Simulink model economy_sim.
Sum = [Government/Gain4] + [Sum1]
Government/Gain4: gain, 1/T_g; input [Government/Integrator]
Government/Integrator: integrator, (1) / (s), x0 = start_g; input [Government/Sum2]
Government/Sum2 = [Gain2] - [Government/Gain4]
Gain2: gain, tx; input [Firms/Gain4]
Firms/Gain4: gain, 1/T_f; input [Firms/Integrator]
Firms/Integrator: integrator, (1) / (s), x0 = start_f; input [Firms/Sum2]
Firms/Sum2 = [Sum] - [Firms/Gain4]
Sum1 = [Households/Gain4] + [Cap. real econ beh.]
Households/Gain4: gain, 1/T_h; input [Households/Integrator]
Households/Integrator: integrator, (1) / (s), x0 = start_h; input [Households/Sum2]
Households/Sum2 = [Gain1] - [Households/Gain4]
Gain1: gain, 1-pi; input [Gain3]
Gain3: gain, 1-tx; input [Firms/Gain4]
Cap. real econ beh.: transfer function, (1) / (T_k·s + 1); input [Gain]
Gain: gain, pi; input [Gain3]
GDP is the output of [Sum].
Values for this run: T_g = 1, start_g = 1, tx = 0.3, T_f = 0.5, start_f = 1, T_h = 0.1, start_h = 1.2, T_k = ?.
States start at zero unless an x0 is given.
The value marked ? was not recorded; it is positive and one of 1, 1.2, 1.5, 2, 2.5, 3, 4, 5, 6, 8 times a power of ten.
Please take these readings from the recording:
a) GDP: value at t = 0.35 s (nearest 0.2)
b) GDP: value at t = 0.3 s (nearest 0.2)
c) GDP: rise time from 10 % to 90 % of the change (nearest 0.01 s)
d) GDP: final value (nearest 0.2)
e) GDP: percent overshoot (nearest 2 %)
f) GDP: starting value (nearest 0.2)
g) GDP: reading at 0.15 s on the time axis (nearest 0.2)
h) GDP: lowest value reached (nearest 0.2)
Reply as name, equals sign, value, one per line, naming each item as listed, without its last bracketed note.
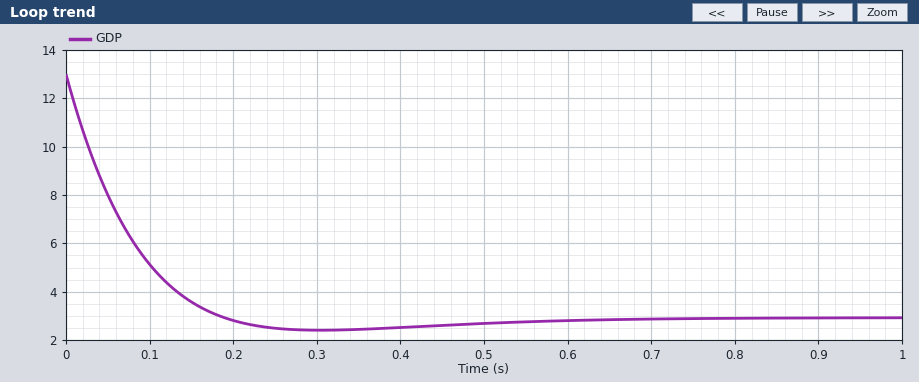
GDP: value at t = 0.35 s = 2.4
GDP: value at t = 0.3 s = 2.4
GDP: rise time from 10 % to 90 % of the change = 0.13 s
GDP: final value = 3.0
GDP: percent overshoot = 6 %
GDP: starting value = 13.0
GDP: reading at 0.15 s on the time axis = 3.6
GDP: lowest value reached = 2.4
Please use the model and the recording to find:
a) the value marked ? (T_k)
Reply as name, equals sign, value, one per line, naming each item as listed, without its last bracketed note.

the value marked ? = 0.2
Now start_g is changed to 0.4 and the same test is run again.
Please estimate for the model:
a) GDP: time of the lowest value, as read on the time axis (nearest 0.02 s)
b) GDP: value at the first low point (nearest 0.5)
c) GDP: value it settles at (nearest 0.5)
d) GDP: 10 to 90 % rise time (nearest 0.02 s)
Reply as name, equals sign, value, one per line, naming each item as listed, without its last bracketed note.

GDP: time of the lowest value, as read on the time axis = 0.30 s
GDP: value at the first low point = 2.0
GDP: value it settles at = 2.5
GDP: 10 to 90 % rise time = 0.12 s
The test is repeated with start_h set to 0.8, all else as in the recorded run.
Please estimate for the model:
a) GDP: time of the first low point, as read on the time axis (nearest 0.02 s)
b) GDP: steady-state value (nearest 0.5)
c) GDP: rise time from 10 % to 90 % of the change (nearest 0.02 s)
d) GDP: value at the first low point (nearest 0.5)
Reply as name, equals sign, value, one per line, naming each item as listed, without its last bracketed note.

GDP: time of the first low point, as read on the time axis = 0.28 s
GDP: steady-state value = 2.5
GDP: rise time from 10 % to 90 % of the change = 0.12 s
GDP: value at the first low point = 2.0
